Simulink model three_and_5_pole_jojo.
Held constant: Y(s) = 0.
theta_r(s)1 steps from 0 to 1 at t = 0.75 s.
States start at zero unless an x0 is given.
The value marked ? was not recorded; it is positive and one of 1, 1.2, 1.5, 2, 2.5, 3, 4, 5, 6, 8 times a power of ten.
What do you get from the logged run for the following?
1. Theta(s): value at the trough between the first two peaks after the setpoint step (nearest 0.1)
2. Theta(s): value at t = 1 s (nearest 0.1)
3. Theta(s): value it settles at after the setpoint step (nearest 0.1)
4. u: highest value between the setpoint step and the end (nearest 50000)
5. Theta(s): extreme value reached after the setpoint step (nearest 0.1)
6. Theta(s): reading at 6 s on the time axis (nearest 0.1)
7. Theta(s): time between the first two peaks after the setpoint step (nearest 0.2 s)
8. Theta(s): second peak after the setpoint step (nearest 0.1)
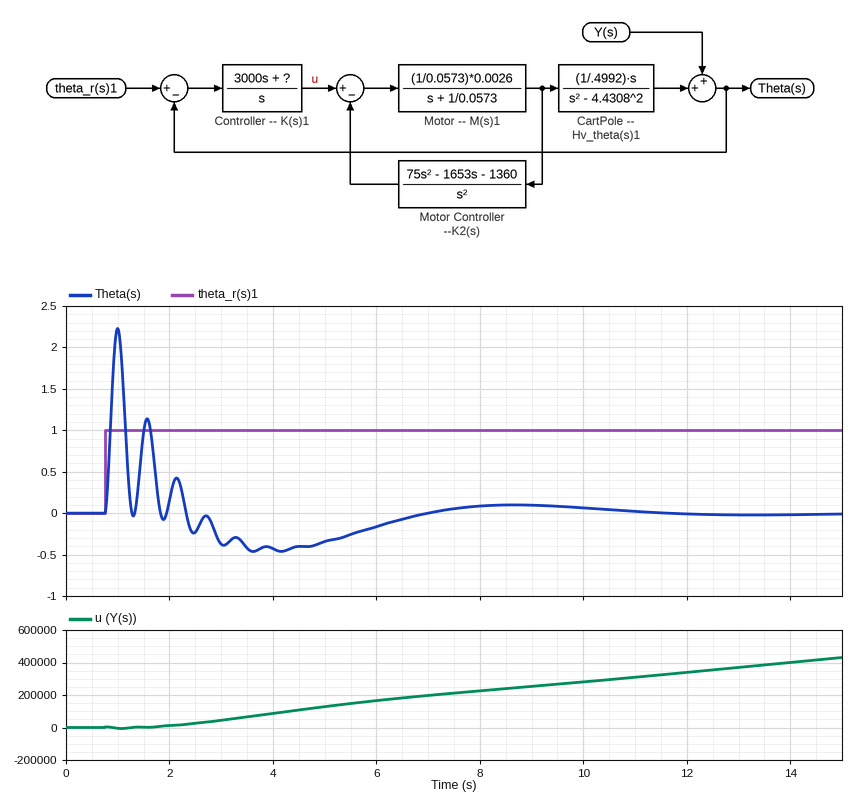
0.0
2.2
0.0
450000
2.2
-0.2
0.6 s
1.1
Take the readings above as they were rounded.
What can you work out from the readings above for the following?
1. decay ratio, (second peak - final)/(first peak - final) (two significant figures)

0.50
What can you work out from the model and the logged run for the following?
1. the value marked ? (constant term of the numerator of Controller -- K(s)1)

30000
